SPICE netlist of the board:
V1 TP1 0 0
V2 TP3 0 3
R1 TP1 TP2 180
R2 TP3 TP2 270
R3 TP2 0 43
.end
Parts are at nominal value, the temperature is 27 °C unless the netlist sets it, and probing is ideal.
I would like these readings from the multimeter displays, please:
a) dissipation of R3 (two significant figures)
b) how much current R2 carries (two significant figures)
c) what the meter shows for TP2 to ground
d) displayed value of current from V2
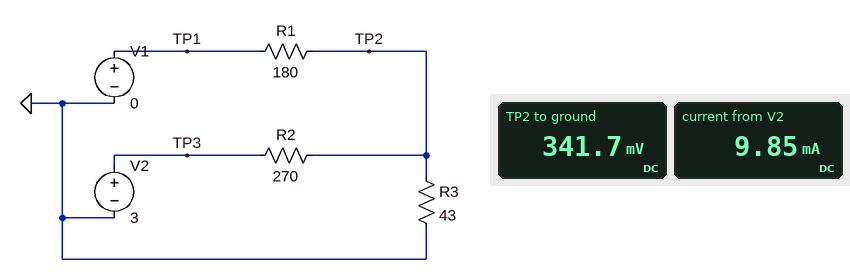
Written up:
2.7 mW
9.8 mA
341.7 mV
9.85 mA
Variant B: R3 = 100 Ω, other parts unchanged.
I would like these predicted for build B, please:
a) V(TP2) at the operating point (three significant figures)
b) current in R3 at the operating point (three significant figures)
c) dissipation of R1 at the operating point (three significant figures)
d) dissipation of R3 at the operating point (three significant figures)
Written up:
577 mV
5.77 mA
1.85 mW
3.33 mW
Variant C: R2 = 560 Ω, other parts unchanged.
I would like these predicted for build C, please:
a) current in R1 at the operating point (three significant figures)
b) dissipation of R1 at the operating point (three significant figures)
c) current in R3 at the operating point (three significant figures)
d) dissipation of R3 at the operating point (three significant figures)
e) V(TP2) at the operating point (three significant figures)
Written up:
973 µA
170 µW
4.07 mA
713 µW
175 mV
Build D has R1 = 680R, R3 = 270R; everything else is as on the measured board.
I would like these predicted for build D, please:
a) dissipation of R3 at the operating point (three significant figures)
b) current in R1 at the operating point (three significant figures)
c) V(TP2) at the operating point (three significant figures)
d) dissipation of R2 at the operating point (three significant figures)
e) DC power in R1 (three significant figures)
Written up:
5.80 mW
1.84 mA
1.25 V
11.3 mW
2.30 mW
